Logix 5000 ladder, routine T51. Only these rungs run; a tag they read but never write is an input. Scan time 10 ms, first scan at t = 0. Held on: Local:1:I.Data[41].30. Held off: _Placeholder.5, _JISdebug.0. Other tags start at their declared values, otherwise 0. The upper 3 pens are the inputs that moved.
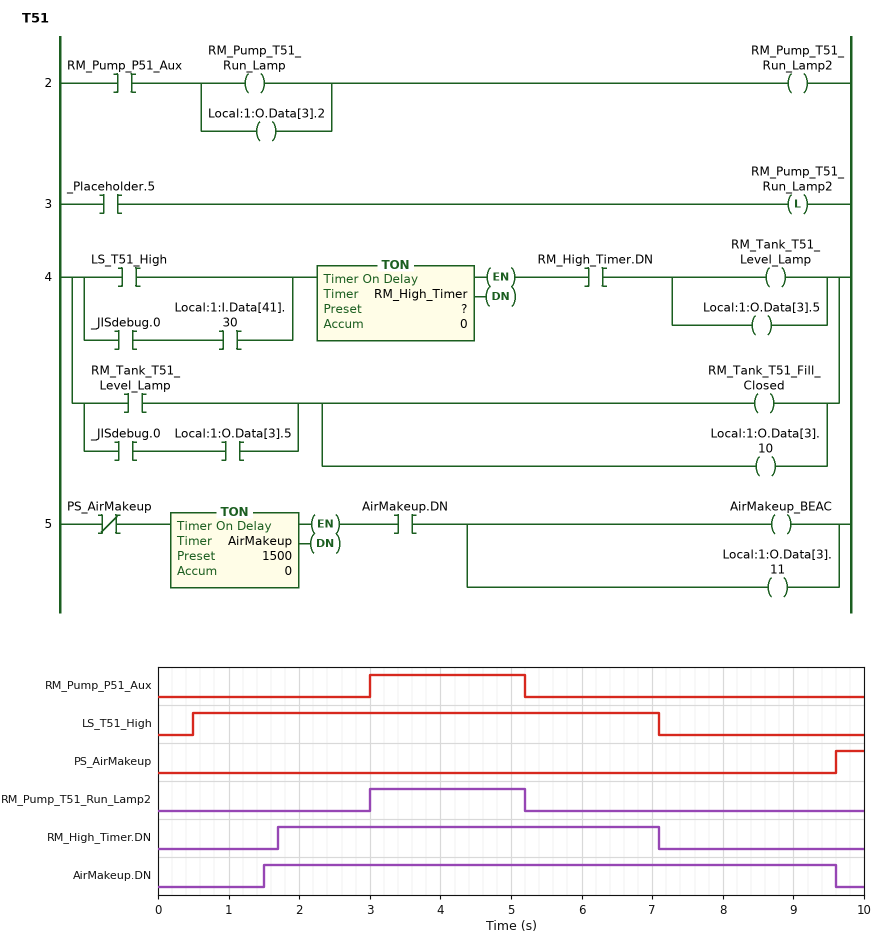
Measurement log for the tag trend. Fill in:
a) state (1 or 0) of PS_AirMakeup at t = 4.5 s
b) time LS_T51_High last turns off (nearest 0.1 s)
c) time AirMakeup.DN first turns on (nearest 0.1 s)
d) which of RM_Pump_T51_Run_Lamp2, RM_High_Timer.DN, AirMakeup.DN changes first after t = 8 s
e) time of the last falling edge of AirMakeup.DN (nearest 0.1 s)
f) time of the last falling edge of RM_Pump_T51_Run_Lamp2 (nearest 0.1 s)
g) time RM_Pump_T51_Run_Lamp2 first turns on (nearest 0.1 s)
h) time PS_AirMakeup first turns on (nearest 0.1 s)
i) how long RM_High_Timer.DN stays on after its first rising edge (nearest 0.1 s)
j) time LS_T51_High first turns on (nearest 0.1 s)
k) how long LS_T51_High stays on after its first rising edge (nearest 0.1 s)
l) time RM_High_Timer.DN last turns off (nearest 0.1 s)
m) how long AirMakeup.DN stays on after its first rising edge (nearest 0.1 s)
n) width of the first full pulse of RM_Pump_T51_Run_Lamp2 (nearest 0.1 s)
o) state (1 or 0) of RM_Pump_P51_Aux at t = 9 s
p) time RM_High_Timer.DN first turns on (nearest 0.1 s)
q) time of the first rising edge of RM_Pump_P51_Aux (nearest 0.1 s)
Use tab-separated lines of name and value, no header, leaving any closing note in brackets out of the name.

state (1 or 0) of PS_AirMakeup at t = 4.5 s	0
time LS_T51_High last turns off	7.1 s
time AirMakeup.DN first turns on	1.5 s
which of RM_Pump_T51_Run_Lamp2, RM_High_Timer.DN, AirMakeup.DN changes first after t = 8 s	AirMakeup.DN
time of the last falling edge of AirMakeup.DN	9.6 s
time of the last falling edge of RM_Pump_T51_Run_Lamp2	5.2 s
time RM_Pump_T51_Run_Lamp2 first turns on	3.0 s
time PS_AirMakeup first turns on	9.6 s
how long RM_High_Timer.DN stays on after its first rising edge	5.4 s
time LS_T51_High first turns on	0.5 s
how long LS_T51_High stays on after its first rising edge	6.6 s
time RM_High_Timer.DN last turns off	7.1 s
how long AirMakeup.DN stays on after its first rising edge	8.1 s
width of the first full pulse of RM_Pump_T51_Run_Lamp2	2.2 s
state (1 or 0) of RM_Pump_P51_Aux at t = 9 s	0
time RM_High_Timer.DN first turns on	1.7 s
time of the first rising edge of RM_Pump_P51_Aux	3.0 s
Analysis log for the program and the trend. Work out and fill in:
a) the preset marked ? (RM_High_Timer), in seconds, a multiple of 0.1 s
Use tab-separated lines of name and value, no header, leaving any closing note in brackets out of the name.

the preset marked ? (RM_High_Timer), in seconds, a multiple of 0.1 s	1.2 s
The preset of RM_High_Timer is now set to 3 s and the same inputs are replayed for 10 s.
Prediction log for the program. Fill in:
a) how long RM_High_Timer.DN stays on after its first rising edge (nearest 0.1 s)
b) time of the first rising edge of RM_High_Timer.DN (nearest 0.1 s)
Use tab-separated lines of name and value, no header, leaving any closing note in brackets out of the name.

how long RM_High_Timer.DN stays on after its first rising edge	3.6 s
time of the first rising edge of RM_High_Timer.DN	3.5 s
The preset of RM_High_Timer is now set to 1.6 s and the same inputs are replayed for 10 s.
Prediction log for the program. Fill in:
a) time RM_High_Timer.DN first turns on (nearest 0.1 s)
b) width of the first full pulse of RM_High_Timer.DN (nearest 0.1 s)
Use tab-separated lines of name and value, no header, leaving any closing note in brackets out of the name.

time RM_High_Timer.DN first turns on	2.1 s
width of the first full pulse of RM_High_Timer.DN	5.0 s
